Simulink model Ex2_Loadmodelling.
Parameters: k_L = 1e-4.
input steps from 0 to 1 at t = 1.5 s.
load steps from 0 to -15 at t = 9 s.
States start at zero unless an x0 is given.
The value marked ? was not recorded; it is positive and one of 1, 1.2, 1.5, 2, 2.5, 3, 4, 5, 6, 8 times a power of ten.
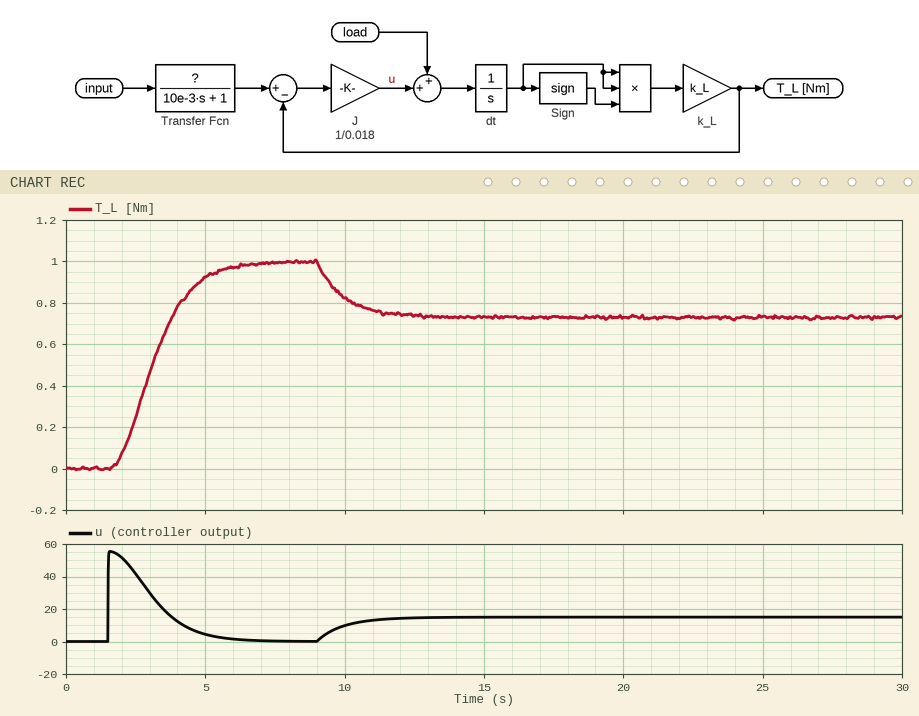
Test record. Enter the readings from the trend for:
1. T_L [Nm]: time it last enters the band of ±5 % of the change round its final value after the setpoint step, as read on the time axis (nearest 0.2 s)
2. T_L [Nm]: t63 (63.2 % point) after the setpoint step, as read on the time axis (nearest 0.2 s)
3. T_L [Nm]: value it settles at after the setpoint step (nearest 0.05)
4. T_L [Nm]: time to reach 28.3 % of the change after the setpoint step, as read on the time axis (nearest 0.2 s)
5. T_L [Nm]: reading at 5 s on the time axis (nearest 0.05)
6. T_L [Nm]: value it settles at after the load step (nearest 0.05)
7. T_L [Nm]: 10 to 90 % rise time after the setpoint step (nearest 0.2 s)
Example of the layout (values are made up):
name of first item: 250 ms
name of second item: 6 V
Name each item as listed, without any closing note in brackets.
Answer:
T_L [Nm]: time it last enters the band of ±5 % of the change round its final value after the setpoint step, as read on the time axis: 5.4 s
T_L [Nm]: t63 (63.2 % point) after the setpoint step, as read on the time axis: 3.4 s
T_L [Nm]: value it settles at after the setpoint step: 1.00
T_L [Nm]: time to reach 28.3 % of the change after the setpoint step, as read on the time axis: 2.6 s
T_L [Nm]: reading at 5 s on the time axis: 0.90
T_L [Nm]: value it settles at after the load step: 0.75
T_L [Nm]: 10 to 90 % rise time after the setpoint step: 2.6 s
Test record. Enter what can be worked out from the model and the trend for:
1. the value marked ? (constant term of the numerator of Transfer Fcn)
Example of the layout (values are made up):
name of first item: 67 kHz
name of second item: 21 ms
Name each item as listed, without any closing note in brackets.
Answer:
the value marked ?: 1
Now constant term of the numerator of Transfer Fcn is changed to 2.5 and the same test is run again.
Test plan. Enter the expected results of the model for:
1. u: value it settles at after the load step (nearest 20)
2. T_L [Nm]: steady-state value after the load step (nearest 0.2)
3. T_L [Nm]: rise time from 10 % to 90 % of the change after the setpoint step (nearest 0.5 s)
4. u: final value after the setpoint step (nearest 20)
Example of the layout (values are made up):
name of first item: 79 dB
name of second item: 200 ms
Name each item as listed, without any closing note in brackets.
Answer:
u: value it settles at after the load step: 20
T_L [Nm]: steady-state value after the load step: 2.2
T_L [Nm]: rise time from 10 % to 90 % of the change after the setpoint step: 1.5 s
u: final value after the setpoint step: 0
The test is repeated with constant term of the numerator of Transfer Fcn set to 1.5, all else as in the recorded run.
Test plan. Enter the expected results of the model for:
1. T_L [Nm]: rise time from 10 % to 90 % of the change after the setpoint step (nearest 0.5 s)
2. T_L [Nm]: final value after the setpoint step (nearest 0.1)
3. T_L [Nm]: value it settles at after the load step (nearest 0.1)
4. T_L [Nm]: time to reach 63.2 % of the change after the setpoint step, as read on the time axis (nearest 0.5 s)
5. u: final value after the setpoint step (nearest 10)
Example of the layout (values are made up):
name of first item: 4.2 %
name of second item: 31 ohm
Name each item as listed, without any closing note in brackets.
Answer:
T_L [Nm]: rise time from 10 % to 90 % of the change after the setpoint step: 2.0 s
T_L [Nm]: final value after the setpoint step: 1.5
T_L [Nm]: value it settles at after the load step: 1.2
T_L [Nm]: time to reach 63.2 % of the change after the setpoint step, as read on the time axis: 3.0 s
u: final value after the setpoint step: 0
